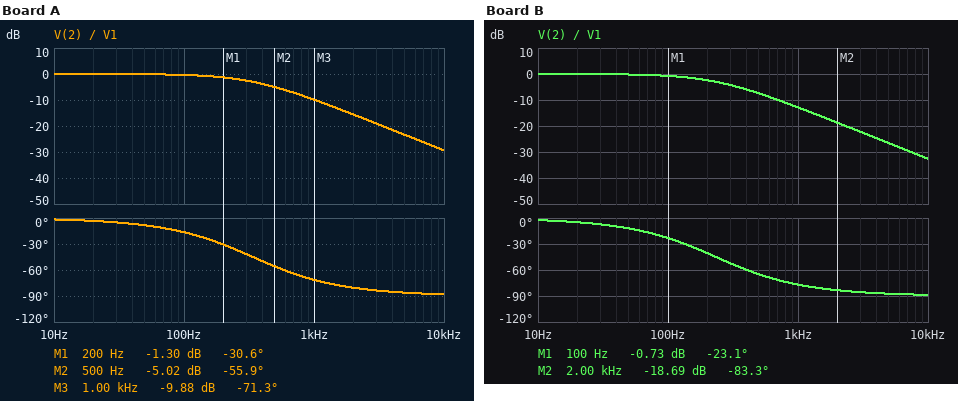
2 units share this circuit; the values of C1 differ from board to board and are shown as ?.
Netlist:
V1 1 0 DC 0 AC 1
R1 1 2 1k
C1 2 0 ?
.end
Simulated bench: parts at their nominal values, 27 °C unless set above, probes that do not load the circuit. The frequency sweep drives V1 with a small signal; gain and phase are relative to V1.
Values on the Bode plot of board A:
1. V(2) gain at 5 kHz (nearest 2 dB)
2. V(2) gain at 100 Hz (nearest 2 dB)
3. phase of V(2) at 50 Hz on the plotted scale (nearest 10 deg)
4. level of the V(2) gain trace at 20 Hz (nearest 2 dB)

-24 dB
0 dB
-10 deg
0 dB
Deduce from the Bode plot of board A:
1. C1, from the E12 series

470 nF
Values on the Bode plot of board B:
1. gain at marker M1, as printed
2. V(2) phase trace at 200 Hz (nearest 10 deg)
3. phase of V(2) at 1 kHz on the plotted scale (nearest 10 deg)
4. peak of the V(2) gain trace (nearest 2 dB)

-0.73 dB
-40 deg
-80 deg
0 dB
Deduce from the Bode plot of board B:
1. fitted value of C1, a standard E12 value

680 nF
